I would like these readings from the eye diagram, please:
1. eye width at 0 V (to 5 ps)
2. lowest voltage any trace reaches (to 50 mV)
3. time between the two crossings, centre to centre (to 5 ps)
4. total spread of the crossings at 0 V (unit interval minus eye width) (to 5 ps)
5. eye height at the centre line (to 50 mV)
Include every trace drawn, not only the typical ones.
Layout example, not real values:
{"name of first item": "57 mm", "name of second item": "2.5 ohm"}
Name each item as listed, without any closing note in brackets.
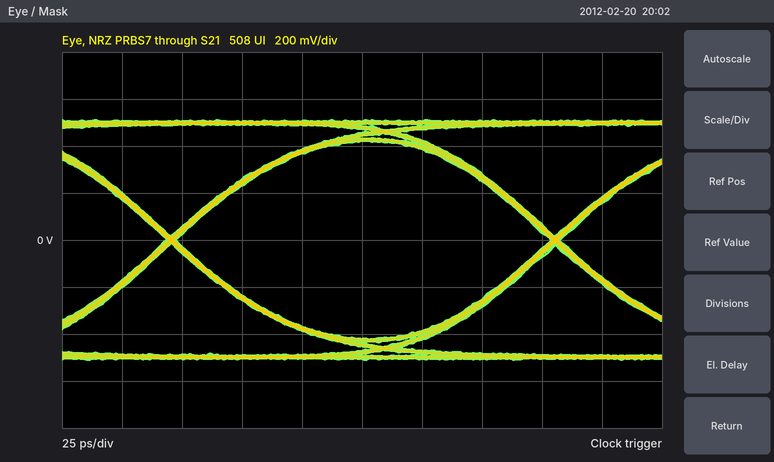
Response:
{"eye width at 0 V": "155 ps", "lowest voltage any trace reaches": "-500 mV", "time between the two crossings, centre to centre": "160 ps", "total spread of the crossings at 0 V (unit interval minus eye width)": "5 ps", "eye height at the centre line": "850 mV"}
